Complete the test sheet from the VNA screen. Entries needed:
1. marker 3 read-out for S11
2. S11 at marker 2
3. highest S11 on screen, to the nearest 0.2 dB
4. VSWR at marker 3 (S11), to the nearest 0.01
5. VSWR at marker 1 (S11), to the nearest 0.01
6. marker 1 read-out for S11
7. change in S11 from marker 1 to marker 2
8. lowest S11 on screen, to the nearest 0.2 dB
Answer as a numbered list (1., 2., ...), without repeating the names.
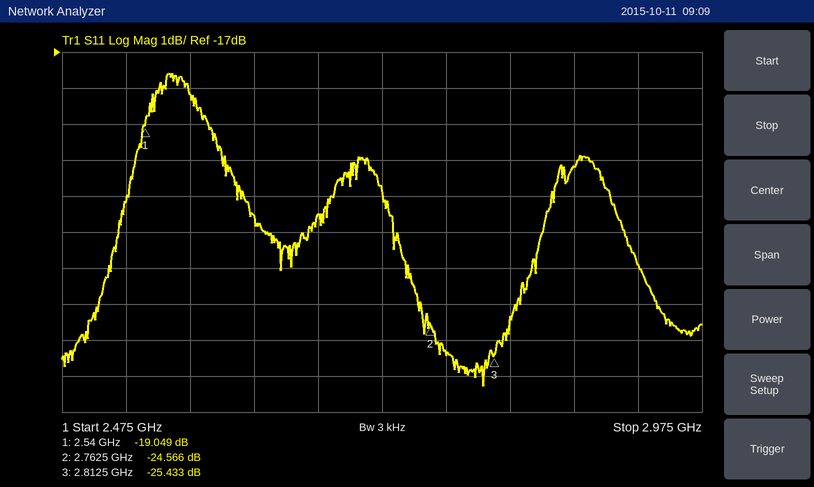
1. -25.433 dB
2. -24.566 dB
3. -17.6 dB
4. 1.11
5. 1.25
6. -19.049 dB
7. -5.517 dB
8. -26.2 dB
